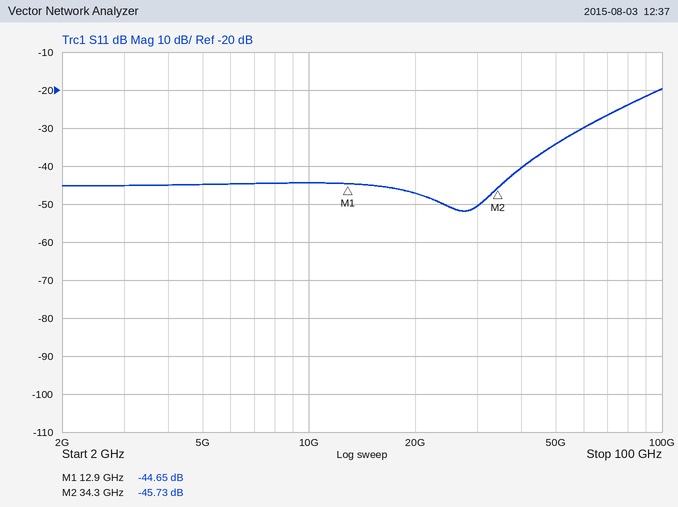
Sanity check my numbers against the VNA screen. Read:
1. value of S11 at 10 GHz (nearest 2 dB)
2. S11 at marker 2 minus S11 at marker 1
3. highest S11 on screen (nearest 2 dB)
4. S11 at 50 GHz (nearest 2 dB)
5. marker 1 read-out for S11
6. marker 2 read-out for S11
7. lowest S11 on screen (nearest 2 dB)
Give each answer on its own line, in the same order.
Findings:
-44 dB
-1.08 dB
-20 dB
-34 dB
-44.65 dB
-45.73 dB
-52 dB
